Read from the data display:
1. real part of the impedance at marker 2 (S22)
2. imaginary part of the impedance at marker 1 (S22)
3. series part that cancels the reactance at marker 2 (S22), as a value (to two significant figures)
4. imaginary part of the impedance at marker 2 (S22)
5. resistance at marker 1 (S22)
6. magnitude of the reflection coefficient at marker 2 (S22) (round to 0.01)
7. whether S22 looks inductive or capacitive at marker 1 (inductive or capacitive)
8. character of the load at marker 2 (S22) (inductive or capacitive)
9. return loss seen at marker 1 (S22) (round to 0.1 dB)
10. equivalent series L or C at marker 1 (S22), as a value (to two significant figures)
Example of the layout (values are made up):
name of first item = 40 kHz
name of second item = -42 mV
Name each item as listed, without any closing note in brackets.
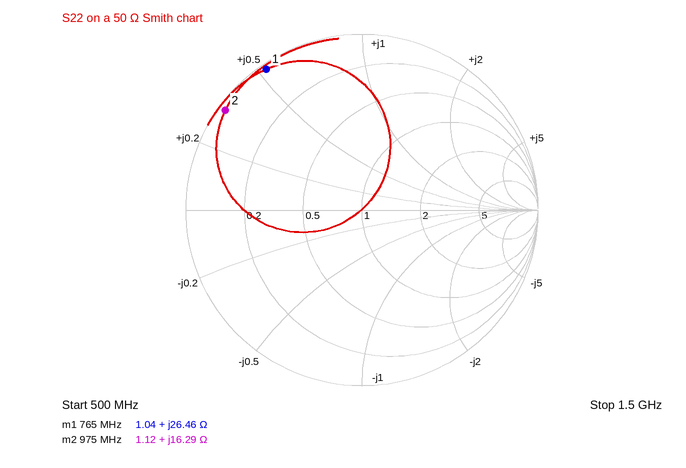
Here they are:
real part of the impedance at marker 2 = 1.12 Ω
imaginary part of the impedance at marker 1 = +26.46 Ω
series part that cancels the reactance at marker 2 (S22), as a value = 10 pF
imaginary part of the impedance at marker 2 = +16.29 Ω
resistance at marker 1 = 1.04 Ω
magnitude of the reflection coefficient at marker 2 (S22) = 0.96
whether S22 looks inductive or capacitive at marker 1 = inductive
character of the load at marker 2 (S22) = inductive
return loss seen at marker 1 (S22) = 0.3 dB
equivalent series L or C at marker 1 (S22), as a value = 5.5 nH
